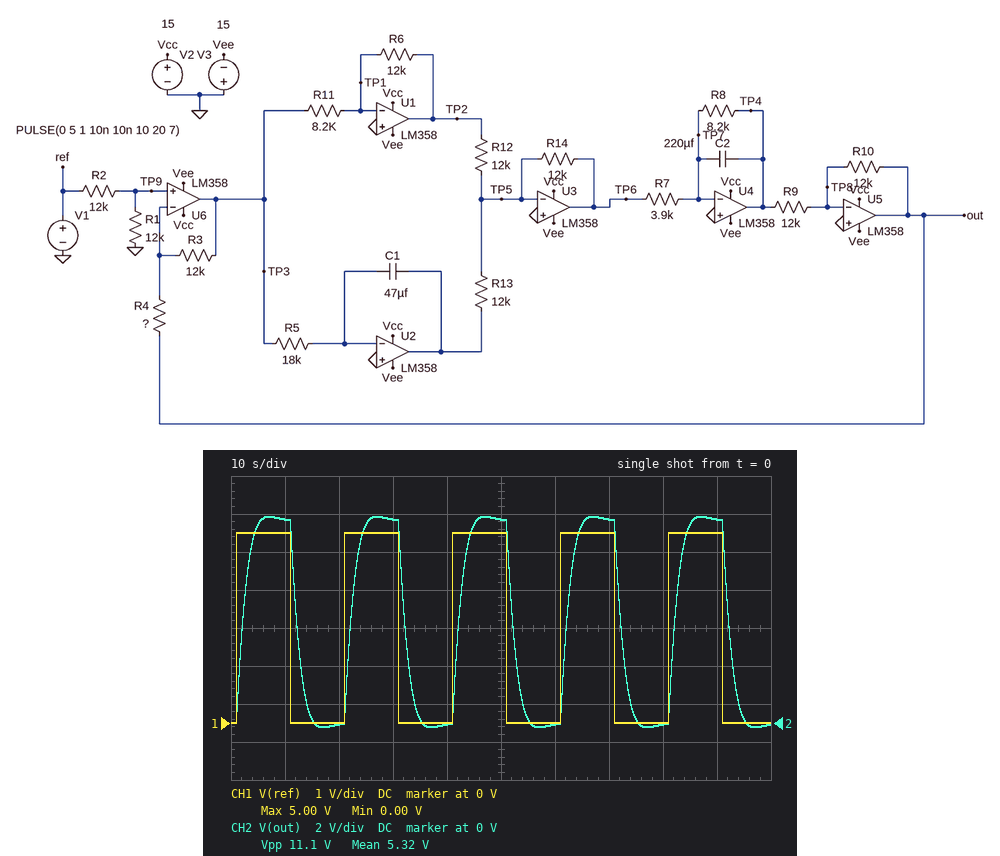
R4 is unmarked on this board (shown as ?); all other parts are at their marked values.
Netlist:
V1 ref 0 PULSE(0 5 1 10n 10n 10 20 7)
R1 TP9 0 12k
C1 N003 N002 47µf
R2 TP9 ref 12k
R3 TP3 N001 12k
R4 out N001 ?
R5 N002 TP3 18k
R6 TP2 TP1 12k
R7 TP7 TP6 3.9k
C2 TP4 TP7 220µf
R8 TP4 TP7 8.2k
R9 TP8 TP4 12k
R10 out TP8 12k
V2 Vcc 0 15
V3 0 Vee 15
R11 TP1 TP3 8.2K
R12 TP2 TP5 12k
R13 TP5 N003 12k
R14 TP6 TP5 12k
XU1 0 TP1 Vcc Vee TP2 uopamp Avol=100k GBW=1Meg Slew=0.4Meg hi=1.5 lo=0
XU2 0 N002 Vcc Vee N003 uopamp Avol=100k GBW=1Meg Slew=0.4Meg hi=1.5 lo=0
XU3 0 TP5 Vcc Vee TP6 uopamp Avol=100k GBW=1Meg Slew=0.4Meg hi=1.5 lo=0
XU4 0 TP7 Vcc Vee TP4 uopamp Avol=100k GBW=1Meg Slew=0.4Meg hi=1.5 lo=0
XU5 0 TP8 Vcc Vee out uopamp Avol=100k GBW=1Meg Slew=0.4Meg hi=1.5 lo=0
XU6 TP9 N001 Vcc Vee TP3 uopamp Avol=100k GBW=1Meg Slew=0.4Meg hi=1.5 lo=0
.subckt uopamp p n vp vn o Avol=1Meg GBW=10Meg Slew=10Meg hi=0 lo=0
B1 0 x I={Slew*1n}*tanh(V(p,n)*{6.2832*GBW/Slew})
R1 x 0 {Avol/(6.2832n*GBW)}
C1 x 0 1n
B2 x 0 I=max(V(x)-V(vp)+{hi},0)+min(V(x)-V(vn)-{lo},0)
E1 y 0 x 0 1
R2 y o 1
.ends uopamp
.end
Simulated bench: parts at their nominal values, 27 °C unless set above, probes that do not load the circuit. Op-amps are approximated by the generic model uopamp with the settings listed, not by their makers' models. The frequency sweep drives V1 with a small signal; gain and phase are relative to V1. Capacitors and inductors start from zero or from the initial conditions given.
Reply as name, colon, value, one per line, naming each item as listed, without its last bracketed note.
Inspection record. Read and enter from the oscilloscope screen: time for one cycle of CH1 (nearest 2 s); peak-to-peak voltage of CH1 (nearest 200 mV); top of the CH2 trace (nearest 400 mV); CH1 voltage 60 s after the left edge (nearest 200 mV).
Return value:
time for one cycle of CH1: 20 s
peak-to-peak voltage of CH1: 5.0 V
top of the CH2 trace: 10.8 V
CH1 voltage 60 s after the left edge: 0 V
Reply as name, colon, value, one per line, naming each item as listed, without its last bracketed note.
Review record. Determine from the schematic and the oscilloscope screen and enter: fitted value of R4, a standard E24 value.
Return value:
fitted value of R4, a standard E24 value: 39 kΩ
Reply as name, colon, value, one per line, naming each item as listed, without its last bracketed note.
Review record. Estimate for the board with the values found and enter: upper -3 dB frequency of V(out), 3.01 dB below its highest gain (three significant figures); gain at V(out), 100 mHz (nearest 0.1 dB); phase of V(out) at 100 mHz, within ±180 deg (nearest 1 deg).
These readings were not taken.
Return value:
upper -3 dB frequency of V(out), 3.01 dB below its highest gain: 119 mHz
gain at V(out), 100 mHz: 4.5 dB
phase of V(out) at 100 mHz, within ±180 deg: -50 deg
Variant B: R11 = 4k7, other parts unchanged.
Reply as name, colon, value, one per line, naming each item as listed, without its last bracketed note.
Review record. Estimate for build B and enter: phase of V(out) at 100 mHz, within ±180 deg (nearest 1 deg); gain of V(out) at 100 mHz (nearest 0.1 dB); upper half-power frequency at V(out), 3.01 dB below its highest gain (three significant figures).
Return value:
phase of V(out) at 100 mHz, within ±180 deg: -35 deg
gain of V(out) at 100 mHz: 4.3 dB
upper half-power frequency at V(out), 3.01 dB below its highest gain: 128 mHz
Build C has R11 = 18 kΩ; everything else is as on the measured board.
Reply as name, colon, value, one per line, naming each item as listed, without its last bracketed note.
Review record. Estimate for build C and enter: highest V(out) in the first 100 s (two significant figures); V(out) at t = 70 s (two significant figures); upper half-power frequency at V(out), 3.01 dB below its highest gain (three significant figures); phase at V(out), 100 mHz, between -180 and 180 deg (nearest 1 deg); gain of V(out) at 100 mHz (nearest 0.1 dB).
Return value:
highest V(out) in the first 100 s: 12 V
V(out) at t = 70 s: 11 V
upper half-power frequency at V(out), 3.01 dB below its highest gain: 120 mHz
phase at V(out), 100 mHz, between -180 and 180 deg: -67 deg
gain of V(out) at 100 mHz: 5.6 dB
